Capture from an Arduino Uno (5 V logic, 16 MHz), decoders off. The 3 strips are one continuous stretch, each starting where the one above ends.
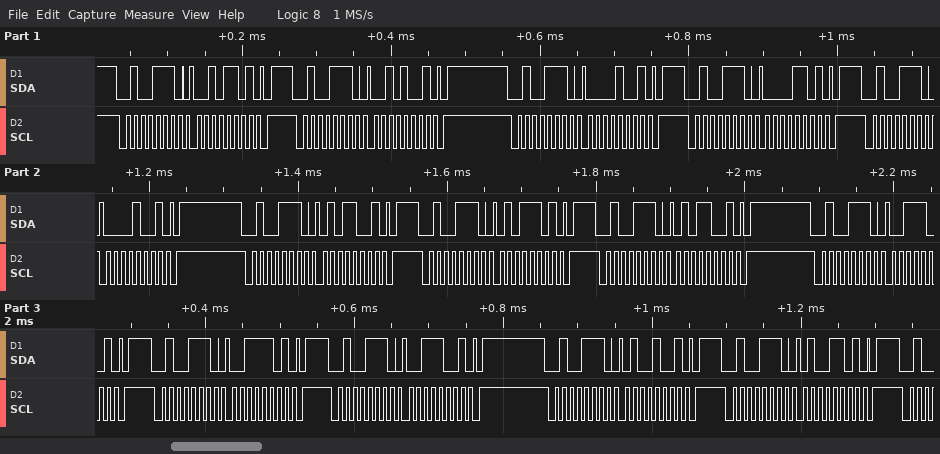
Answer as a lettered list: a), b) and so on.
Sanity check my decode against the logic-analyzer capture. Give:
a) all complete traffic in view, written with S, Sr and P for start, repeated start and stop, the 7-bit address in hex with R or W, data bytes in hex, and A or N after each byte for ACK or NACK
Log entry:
a) S 27W A 2D A P S 27W A 29 A P S 27W A 09 A P S 27W A 0D A P S 27W A 09 A P S 27W A 59 A P S 27W A 5D A P S 27W A 59 A P S 27W A 39 A P S 27W A 3D A P S 27W A 39 A P S 27W A 49 A P S 27W A 4D A P
